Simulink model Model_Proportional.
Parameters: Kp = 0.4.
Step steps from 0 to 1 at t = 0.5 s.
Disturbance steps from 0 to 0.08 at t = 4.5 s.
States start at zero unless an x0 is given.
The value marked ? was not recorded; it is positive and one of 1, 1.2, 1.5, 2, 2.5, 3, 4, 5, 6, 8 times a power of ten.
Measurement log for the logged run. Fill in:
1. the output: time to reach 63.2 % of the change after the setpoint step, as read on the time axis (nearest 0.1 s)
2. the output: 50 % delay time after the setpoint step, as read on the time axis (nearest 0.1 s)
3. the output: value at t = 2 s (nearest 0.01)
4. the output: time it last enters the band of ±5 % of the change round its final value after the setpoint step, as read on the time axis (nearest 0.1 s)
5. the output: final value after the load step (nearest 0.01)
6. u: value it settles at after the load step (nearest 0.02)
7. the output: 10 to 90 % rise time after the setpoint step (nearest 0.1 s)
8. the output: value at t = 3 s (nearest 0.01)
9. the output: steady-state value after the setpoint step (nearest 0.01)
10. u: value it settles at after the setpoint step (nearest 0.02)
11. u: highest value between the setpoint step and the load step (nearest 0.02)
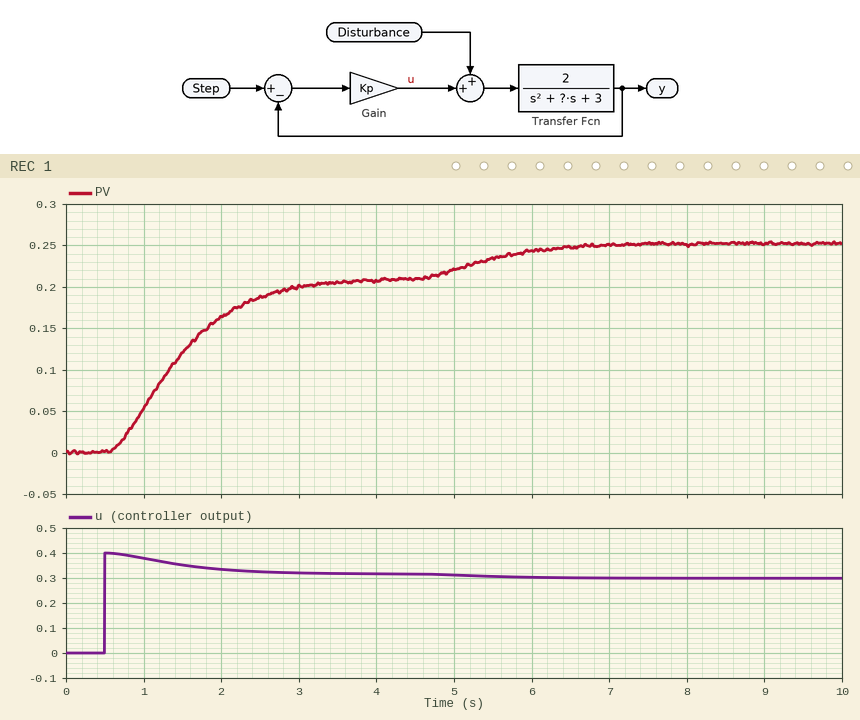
1.6 s
1.4 s
0.16
3.0 s
0.25
0.30
1.8 s
0.20
0.21
0.32
0.40
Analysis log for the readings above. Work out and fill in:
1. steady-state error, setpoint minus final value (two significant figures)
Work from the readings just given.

0.79
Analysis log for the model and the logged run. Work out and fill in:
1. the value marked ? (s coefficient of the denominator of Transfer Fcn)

4
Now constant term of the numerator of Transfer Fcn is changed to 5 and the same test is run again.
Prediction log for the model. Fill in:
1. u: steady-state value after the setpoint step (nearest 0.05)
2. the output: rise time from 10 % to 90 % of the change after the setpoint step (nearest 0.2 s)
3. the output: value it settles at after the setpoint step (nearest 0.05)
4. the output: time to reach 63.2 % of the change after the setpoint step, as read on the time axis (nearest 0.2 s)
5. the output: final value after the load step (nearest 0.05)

0.25
1.2 s
0.40
1.4 s
0.50
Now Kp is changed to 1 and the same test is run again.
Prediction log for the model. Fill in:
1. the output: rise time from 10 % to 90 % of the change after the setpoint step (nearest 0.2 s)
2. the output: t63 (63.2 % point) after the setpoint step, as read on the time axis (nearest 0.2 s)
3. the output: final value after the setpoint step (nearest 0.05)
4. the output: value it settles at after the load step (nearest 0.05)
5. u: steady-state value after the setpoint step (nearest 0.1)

1.2 s
1.4 s
0.40
0.45
0.6
